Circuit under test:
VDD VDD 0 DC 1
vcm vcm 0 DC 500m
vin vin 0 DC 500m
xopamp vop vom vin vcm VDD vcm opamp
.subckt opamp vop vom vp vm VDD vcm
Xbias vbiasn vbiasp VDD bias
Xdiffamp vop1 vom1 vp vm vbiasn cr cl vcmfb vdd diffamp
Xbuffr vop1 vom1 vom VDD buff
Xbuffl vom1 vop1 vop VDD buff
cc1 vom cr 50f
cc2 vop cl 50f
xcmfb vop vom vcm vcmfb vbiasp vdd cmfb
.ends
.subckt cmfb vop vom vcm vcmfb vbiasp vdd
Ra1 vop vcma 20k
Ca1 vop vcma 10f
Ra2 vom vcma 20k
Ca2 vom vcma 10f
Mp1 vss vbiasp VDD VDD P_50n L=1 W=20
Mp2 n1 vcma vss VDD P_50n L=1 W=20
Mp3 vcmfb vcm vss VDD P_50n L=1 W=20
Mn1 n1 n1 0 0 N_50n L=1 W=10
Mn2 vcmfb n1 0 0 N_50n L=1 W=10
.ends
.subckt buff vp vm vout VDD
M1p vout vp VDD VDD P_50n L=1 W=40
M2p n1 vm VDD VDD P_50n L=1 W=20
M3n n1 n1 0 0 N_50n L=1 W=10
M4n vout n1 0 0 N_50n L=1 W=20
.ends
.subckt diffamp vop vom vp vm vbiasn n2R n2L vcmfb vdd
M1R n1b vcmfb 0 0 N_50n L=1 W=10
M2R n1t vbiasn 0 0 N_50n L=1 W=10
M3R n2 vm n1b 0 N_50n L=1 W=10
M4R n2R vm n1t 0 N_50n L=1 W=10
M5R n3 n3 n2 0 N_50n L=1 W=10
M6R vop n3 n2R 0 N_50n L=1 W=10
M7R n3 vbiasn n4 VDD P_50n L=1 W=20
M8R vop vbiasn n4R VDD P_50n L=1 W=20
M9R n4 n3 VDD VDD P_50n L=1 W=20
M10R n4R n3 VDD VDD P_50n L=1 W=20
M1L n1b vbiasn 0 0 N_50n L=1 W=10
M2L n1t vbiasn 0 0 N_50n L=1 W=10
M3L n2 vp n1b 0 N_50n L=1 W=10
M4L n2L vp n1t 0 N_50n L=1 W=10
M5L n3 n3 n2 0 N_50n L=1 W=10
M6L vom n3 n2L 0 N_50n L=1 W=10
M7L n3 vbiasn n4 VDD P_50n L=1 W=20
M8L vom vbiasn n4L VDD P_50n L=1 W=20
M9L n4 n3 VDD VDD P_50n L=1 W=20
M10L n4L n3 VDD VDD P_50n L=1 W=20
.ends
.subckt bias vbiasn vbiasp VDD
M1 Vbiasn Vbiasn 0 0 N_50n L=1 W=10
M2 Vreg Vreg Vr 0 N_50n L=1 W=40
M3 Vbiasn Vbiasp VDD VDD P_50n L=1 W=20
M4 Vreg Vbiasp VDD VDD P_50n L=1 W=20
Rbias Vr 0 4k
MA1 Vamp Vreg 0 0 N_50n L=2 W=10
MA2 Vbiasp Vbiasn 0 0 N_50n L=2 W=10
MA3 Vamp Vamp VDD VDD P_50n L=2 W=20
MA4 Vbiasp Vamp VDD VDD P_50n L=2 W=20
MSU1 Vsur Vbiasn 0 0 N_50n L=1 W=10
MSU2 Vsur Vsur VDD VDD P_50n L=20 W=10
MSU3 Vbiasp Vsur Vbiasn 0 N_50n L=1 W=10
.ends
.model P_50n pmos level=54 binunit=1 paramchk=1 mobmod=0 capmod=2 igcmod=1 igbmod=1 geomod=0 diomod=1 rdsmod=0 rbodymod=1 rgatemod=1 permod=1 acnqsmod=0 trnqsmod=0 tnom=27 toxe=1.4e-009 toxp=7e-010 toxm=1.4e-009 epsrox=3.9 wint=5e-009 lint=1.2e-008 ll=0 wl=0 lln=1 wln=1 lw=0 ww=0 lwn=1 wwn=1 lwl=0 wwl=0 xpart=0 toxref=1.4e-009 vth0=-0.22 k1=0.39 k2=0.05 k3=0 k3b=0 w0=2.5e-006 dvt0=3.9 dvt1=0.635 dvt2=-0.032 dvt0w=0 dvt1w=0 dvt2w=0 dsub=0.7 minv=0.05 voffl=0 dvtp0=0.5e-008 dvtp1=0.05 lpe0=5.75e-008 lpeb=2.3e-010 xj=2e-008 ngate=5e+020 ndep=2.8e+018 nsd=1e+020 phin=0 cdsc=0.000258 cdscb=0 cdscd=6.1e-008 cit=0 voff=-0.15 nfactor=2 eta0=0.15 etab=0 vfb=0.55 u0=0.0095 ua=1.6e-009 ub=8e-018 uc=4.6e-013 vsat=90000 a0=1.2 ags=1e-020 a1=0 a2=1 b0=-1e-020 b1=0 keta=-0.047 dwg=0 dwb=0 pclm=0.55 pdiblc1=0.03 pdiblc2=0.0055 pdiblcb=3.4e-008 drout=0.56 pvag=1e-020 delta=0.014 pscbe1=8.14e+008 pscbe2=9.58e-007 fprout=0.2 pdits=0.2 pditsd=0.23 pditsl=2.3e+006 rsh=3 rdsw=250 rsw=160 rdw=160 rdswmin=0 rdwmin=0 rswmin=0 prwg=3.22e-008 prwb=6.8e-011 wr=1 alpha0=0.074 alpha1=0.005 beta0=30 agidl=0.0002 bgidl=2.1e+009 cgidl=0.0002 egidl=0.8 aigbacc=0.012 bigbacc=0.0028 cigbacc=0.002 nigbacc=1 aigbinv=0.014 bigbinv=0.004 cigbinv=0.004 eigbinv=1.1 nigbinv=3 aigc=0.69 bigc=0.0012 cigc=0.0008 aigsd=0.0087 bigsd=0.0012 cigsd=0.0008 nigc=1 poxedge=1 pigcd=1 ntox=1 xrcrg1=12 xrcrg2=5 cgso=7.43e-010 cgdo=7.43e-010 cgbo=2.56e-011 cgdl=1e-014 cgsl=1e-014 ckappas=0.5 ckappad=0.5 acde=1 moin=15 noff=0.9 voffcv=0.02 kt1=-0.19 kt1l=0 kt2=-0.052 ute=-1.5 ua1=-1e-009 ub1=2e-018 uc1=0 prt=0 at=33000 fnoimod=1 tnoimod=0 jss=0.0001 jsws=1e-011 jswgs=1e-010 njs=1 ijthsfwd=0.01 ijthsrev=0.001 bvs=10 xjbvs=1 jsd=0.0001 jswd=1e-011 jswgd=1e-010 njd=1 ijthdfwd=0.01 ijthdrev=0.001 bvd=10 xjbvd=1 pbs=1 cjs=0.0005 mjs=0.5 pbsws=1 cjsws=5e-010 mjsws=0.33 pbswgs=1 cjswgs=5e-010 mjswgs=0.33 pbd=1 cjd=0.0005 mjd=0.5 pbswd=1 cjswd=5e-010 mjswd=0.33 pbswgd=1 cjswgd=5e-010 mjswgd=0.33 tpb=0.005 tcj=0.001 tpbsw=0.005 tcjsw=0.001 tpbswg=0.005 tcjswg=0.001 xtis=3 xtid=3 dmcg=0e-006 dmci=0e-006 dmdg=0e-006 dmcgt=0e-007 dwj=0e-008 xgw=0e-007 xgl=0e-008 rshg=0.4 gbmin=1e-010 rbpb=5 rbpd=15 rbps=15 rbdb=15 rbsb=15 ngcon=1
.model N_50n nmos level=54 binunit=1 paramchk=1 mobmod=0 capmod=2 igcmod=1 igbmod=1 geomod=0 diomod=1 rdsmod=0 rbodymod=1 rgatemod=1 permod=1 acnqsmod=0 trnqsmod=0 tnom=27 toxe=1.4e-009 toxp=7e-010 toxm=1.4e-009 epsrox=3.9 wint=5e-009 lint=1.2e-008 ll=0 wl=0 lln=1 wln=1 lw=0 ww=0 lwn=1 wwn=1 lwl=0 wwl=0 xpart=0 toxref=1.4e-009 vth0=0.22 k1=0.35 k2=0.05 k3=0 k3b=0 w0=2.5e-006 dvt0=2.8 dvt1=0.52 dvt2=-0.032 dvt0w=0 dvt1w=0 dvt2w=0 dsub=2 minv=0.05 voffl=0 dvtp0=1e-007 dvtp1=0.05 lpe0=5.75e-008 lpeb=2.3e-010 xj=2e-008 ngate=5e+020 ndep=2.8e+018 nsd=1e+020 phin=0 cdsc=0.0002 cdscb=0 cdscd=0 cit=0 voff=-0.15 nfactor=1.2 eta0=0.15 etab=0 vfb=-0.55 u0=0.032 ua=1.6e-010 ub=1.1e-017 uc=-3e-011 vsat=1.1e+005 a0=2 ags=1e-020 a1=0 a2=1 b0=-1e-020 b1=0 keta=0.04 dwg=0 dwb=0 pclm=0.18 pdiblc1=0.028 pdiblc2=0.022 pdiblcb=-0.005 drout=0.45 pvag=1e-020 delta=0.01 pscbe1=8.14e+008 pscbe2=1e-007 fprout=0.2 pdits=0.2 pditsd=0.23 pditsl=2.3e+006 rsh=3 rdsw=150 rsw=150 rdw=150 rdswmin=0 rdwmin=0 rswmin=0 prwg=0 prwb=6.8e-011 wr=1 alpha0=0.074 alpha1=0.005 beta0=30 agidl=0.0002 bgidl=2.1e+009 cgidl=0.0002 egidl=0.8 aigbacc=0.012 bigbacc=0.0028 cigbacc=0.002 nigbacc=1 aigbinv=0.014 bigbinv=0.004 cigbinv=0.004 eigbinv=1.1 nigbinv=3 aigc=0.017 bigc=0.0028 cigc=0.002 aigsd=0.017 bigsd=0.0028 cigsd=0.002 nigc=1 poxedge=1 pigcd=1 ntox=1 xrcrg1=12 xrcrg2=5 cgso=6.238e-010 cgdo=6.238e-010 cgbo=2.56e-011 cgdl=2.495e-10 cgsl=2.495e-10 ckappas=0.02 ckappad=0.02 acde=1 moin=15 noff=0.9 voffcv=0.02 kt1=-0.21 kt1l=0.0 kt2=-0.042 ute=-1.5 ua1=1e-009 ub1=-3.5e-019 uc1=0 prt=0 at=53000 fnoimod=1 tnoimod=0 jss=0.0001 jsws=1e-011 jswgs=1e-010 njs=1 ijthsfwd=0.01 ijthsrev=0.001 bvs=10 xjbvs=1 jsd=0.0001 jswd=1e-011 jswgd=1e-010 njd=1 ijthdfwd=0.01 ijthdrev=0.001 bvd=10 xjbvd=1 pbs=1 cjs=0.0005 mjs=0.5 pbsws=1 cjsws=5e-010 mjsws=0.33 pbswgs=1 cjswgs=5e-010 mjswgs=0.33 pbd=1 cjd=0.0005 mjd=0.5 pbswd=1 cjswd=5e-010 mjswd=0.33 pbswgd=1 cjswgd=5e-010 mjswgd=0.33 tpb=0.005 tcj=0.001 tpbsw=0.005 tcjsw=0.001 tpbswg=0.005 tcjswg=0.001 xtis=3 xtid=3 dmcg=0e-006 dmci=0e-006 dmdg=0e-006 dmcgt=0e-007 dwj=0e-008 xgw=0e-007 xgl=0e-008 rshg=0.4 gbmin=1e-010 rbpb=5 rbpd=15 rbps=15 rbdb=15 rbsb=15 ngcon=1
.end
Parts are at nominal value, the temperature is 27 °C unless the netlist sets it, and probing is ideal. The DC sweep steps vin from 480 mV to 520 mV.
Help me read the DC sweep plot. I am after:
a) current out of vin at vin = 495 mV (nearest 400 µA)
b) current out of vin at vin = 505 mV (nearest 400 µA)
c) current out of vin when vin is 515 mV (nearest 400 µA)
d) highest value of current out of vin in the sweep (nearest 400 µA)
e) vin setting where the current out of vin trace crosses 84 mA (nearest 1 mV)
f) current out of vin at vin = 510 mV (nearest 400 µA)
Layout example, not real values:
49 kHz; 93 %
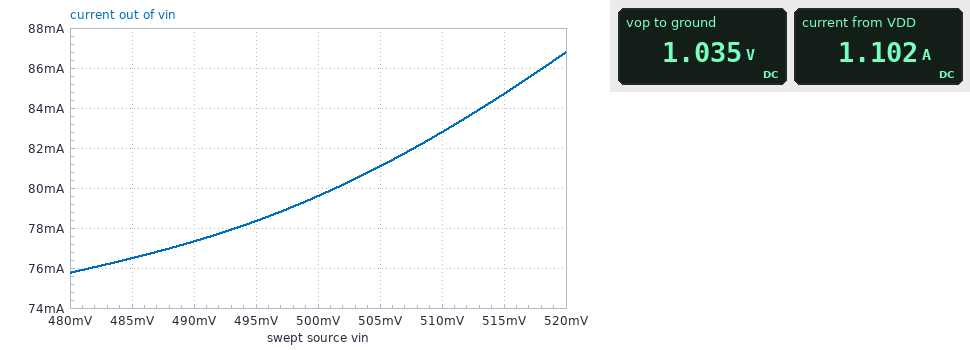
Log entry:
78.4 mA; 81.2 mA; 84.8 mA; 86.8 mA; 513 mV; 82.8 mA
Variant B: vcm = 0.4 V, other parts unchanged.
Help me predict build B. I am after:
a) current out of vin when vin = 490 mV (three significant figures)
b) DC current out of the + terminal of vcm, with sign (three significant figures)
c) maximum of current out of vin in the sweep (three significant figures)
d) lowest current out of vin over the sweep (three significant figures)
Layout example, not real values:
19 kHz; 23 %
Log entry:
78.9 mA; -14.0 mA; 86.2 mA; 77.5 mA
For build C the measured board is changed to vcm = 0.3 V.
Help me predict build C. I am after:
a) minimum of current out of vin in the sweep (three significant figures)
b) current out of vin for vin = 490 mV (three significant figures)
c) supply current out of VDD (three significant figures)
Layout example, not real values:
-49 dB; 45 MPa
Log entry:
78.5 mA; 79.9 mA; 1.13 A
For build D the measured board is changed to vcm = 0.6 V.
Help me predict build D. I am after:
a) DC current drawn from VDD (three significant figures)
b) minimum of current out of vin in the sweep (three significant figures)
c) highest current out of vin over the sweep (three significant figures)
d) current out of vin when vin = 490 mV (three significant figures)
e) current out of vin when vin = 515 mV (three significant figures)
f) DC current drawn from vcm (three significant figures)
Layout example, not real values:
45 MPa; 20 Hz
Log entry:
1.08 A; 77.4 mA; 85.2 mA; 79.1 mA; 83.9 mA; 97.5 mA
